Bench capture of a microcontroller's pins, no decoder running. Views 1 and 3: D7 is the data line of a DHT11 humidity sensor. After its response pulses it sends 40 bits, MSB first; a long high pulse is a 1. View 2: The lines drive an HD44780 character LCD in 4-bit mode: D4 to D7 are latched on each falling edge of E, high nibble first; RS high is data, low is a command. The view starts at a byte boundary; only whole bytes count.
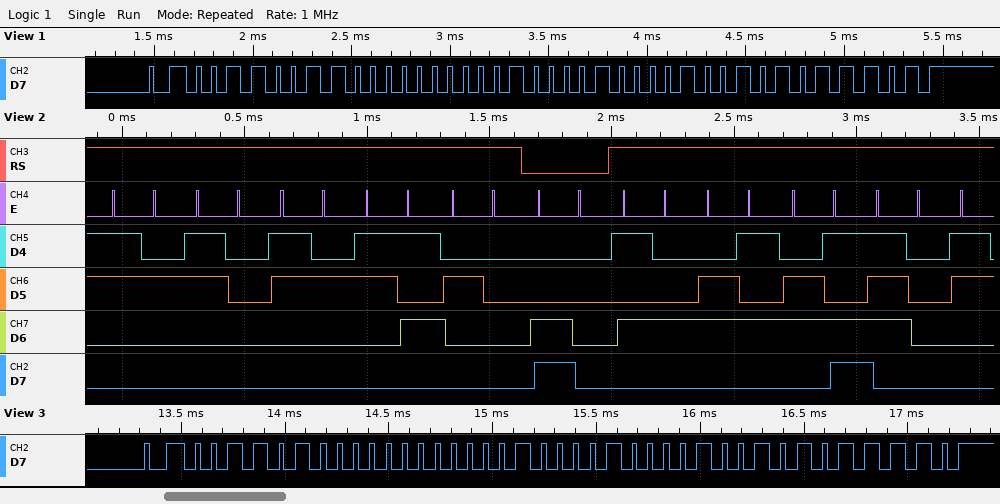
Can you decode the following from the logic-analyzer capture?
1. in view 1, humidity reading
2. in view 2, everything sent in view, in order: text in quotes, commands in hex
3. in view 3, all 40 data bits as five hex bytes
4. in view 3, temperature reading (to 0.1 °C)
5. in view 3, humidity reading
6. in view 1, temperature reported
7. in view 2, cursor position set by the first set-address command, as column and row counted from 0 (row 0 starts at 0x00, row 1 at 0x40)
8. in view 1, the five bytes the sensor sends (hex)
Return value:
51 %
"2025 " 0xC0 "Temp"
34 00 21 09 5E
33.9 °C
52 %
33.9 °C
column 0, row 1
33 00 21 09 5D
